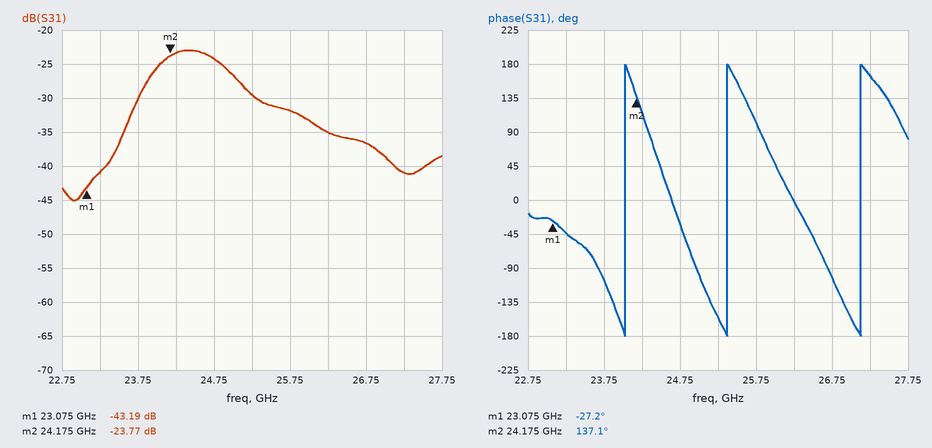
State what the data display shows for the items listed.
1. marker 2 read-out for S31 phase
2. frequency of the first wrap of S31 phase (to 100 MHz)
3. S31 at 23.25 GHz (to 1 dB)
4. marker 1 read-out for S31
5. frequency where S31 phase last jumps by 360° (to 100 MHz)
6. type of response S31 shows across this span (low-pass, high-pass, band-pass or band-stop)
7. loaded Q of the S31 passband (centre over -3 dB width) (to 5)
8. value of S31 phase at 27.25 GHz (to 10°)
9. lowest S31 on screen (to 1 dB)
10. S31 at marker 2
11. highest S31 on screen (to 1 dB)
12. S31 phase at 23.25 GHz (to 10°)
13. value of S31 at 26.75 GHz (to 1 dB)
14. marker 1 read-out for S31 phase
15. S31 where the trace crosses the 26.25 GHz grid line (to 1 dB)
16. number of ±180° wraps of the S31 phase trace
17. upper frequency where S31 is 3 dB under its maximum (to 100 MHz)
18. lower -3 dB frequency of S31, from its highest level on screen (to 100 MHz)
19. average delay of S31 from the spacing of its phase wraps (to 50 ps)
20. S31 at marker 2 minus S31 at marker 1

137.1°
24.0 GHz
-41 dB
-43.19 dB
27.1 GHz
band-pass
25
160°
-45 dB
-23.77 dB
-23 dB
-40°
-37 dB
-27.2°
-35 dB
3
24.9 GHz
24.0 GHz
650 ps
19.42 dB
